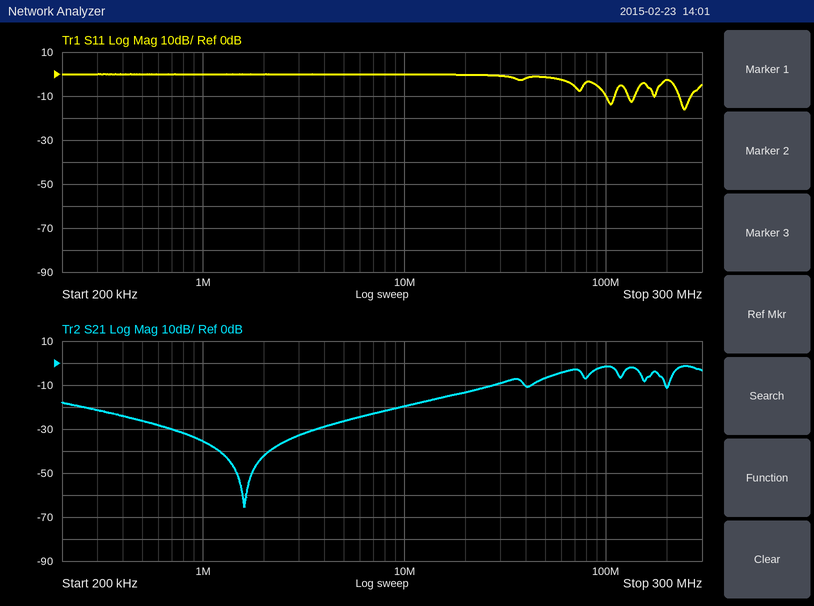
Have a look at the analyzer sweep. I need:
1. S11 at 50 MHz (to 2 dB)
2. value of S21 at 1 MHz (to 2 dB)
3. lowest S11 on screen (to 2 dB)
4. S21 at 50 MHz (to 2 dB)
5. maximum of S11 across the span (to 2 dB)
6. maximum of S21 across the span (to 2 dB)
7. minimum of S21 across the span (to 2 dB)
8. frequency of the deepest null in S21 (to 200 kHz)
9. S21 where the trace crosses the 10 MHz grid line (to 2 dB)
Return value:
-2 dB
-36 dB
-16 dB
-6 dB
0 dB
-2 dB
-66 dB
1.6 MHz
-20 dB
